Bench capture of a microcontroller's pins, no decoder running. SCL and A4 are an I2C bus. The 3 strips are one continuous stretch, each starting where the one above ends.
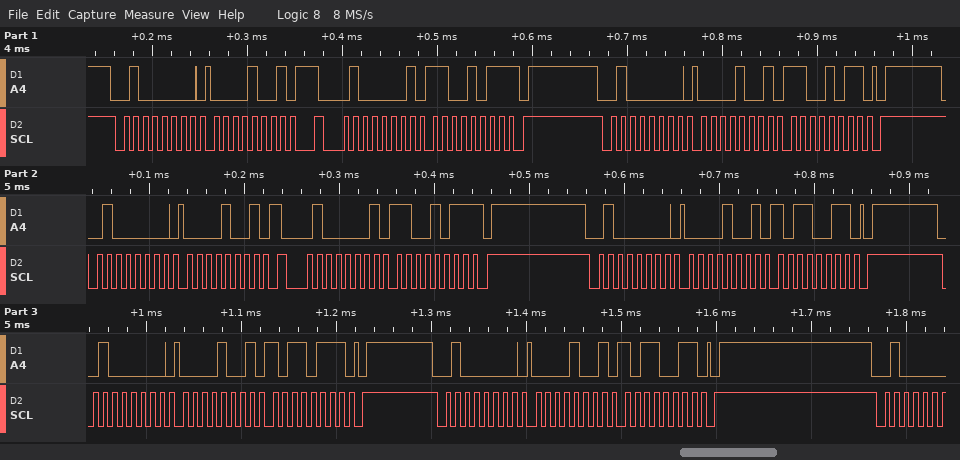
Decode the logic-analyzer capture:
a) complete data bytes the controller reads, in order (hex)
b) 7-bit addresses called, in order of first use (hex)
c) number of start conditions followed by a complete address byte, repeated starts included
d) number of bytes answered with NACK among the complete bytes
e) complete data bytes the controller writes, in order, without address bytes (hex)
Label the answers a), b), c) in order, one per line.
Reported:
a) CB CB
b) 0x20
c) 8
d) 2
e) 09 09 CB 09 09 B3 09 B7 09 B3
